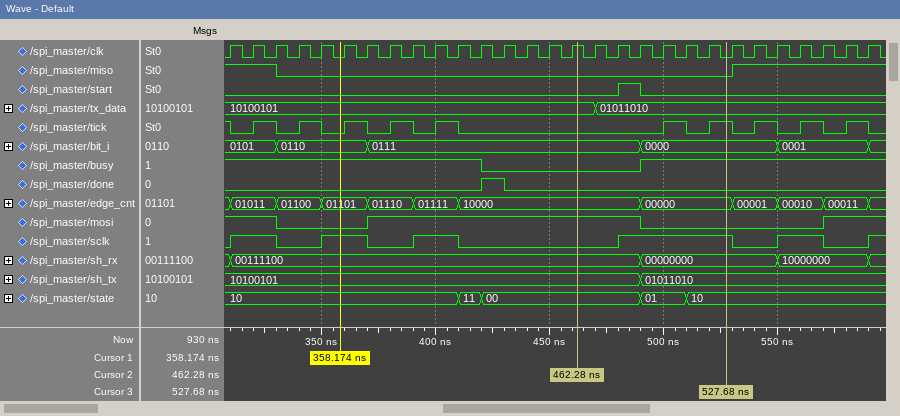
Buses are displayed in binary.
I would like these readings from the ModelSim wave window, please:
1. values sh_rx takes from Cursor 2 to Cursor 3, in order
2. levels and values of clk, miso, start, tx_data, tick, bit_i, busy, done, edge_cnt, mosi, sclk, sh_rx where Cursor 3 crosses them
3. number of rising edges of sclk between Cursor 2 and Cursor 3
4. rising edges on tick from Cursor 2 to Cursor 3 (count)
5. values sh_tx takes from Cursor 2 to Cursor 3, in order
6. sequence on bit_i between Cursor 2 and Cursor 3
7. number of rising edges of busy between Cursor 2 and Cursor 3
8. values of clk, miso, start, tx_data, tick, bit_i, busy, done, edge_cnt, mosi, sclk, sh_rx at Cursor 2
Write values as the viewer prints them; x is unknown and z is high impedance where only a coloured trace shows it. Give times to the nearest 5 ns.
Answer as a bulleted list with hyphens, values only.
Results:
- 00111100, 00000000
- clk=0, miso=0, start=0, tx_data=01011010, tick=1, bit_i=0000, busy=1, done=0, edge_cnt=00000, mosi=0, sclk=1, sh_rx=00000000
- 1
- 2
- 10100101, 01011010
- 0111, 0000
- 1
- clk=1, miso=0, start=0, tx_data=10100101, tick=0, bit_i=0111, busy=0, done=0, edge_cnt=10000, mosi=1, sclk=0, sh_rx=00111100
